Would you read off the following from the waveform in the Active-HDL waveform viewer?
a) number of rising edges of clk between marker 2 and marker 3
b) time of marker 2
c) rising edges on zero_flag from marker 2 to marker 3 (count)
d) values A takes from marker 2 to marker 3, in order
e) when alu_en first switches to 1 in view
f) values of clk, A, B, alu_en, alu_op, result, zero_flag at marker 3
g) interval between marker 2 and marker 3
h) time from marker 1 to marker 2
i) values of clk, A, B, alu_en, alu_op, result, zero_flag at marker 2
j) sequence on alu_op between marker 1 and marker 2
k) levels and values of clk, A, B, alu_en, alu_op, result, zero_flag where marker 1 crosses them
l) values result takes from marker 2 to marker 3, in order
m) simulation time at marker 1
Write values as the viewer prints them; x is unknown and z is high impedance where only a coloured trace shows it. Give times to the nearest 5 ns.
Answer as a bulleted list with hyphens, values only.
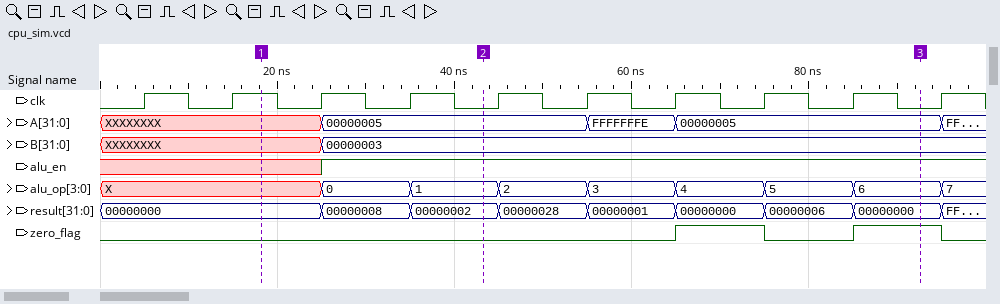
- 5
- 45 ns
- 2
- 00000005, FFFFFFFE, 00000005
- 25 ns
- clk=0, A=00000005, B=00000003, alu_en=1, alu_op=6, result=00000000, zero_flag=1
- 50 ns
- 25 ns
- clk=0, A=00000005, B=00000003, alu_en=1, alu_op=1, result=00000002, zero_flag=0
- X, 0, 1
- clk=1, A=XXXXXXXX, B=XXXXXXXX, alu_en=x, alu_op=X, result=00000000, zero_flag=0
- 00000002, 00000028, 00000001, 00000000, 00000006, 00000000
- 20 ns
